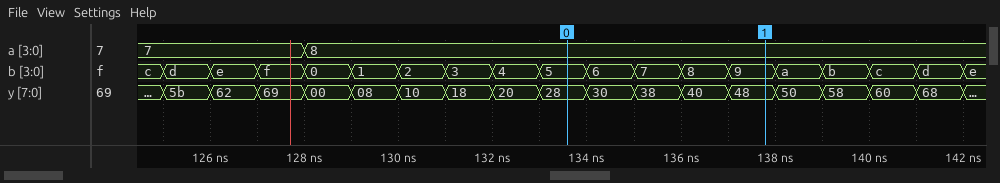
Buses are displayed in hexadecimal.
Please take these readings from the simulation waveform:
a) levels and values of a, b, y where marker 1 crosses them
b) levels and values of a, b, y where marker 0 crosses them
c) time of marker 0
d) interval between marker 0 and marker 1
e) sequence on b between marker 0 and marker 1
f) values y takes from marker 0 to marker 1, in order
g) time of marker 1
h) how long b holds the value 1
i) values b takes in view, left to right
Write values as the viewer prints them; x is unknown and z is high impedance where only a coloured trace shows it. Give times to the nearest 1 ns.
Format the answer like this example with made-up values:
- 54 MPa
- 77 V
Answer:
- a=8, b=9, y=48
- a=8, b=5, y=28
- 134 ns
- 4 ns
- 5, 6, 7, 8, 9
- 28, 30, 38, 40, 48
- 138 ns
- 1 ns
- c, d, e, f, 0, 1, 2, 3, 4, 5, 6, 7, 8, 9, a, b, c, d, e
